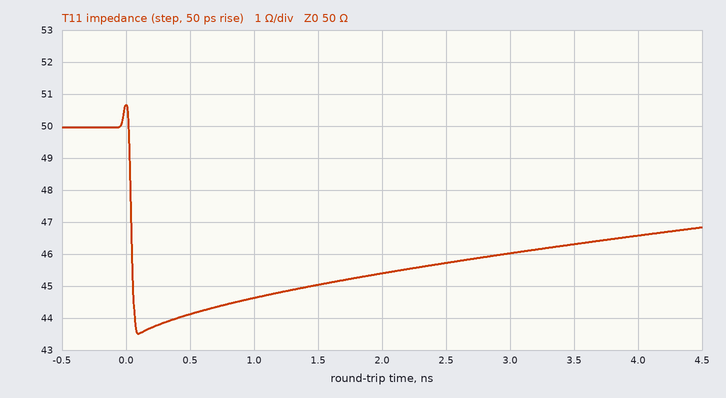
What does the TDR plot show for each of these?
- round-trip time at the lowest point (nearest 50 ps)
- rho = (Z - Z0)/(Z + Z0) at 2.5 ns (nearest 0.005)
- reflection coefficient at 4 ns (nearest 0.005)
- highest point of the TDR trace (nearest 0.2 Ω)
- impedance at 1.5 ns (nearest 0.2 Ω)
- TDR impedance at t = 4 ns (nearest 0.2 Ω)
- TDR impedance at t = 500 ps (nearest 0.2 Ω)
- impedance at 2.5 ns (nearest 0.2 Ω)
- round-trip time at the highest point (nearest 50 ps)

100 ps
-0.045
-0.035
50.6 Ω
45.0 Ω
46.6 Ω
44.2 Ω
45.8 Ω
0 ps
